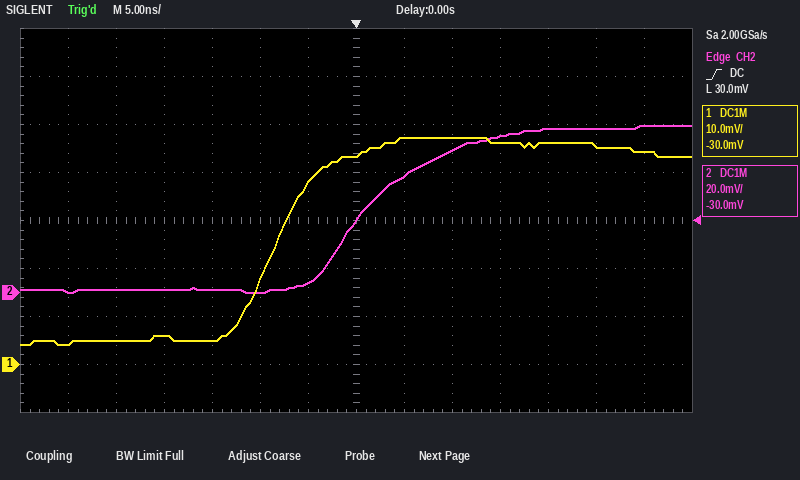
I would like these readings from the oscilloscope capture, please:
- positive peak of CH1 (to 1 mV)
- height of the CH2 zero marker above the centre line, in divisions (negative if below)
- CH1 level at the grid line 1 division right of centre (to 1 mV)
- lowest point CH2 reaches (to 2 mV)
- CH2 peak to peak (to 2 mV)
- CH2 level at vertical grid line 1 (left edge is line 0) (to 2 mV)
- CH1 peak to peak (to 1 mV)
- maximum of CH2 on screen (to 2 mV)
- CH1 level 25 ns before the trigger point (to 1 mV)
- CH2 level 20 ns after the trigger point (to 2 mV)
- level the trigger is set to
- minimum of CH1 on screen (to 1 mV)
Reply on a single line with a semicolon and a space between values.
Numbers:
47 mV; -1.5 div; 47 mV; 0 mV; 70 mV; 0 mV; 43 mV; 70 mV; 5 mV; 68 mV; 30.0 mV; 4 mV
